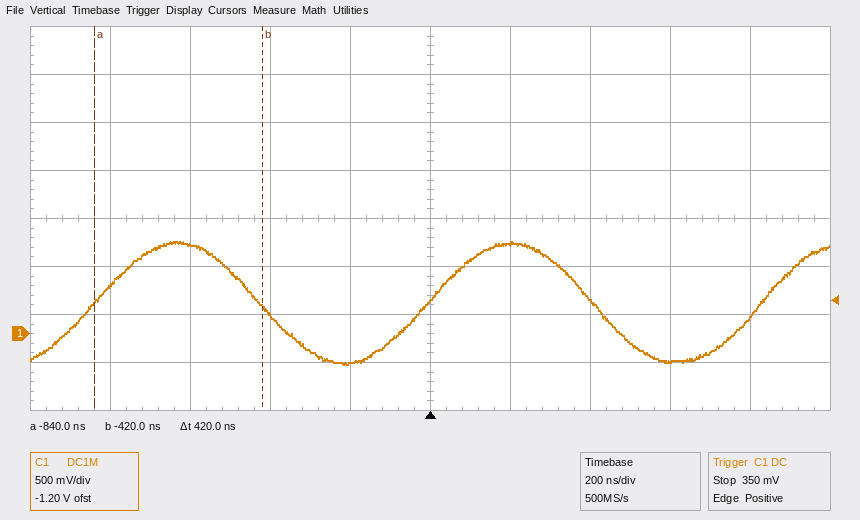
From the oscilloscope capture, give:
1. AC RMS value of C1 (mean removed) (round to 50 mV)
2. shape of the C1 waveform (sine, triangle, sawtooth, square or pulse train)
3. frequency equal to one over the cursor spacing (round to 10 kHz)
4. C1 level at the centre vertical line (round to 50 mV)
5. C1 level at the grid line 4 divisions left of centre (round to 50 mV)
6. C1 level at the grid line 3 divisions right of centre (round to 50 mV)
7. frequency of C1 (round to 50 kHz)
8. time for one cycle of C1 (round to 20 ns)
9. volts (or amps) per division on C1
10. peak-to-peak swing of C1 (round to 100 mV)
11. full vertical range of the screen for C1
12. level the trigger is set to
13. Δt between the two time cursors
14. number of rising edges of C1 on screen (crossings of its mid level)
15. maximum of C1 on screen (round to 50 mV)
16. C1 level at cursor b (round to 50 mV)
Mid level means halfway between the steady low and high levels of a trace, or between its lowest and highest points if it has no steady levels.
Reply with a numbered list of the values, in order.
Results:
1. 450 mV
2. sine
3. 2.38 MHz
4. 350 mV
5. 500 mV
6. -300 mV
7. 1.20 MHz
8. 840 ns
9. 500 mV
10. 1.30 V
11. 4 V
12. 350 mV
13. 420 ns
14. 3
15. 950 mV
16. 300 mV
